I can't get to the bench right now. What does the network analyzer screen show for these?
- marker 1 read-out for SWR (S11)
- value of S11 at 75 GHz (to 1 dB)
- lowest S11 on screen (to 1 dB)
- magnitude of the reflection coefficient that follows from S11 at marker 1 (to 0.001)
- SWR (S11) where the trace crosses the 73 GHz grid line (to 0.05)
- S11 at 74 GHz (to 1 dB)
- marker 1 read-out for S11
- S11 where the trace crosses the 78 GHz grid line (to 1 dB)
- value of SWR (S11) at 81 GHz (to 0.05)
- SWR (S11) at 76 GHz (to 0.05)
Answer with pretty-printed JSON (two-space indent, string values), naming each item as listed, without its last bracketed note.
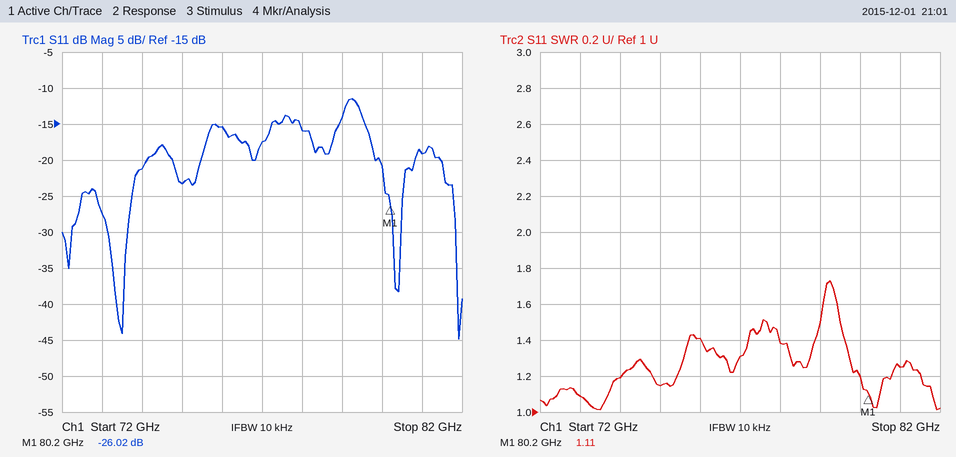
{
  "marker 1 read-out for SWR": "1.11",
  "value of S11 at 75 GHz": "-23 dB",
  "lowest S11 on screen": "-45 dB",
  "magnitude of the reflection coefficient that follows from S11 at marker 1": "0.050",
  "SWR (S11) where the trace crosses the 73 GHz grid line": "1.10",
  "S11 at 74 GHz": "-21 dB",
  "marker 1 read-out for S11": "-26.02 dB",
  "S11 where the trace crosses the 78 GHz grid line": "-16 dB",
  "value of SWR (S11) at 81 GHz": "1.25",
  "SWR (S11) at 76 GHz": "1.40"
}
